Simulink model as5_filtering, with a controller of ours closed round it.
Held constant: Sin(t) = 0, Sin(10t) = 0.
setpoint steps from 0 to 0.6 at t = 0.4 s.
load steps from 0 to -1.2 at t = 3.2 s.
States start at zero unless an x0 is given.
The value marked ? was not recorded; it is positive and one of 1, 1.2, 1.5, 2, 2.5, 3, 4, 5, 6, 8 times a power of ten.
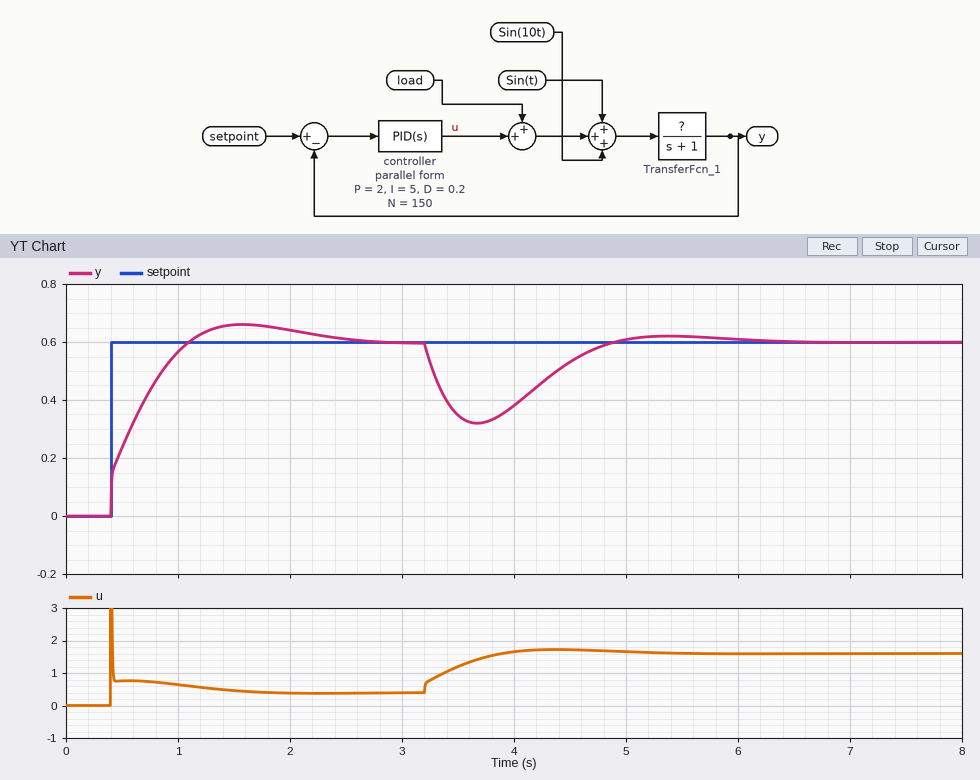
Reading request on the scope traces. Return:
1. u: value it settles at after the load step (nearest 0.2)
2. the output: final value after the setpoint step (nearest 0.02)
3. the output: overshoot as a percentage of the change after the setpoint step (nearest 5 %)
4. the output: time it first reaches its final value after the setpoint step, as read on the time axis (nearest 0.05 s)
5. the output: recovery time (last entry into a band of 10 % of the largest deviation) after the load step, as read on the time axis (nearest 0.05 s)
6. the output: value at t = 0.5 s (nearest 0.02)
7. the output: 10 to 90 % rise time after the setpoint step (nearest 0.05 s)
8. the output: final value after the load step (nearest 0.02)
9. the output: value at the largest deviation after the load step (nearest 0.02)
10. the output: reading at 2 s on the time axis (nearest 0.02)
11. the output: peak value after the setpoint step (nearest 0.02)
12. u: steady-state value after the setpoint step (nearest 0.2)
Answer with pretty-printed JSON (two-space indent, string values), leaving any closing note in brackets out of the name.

{
  "u: value it settles at after the load step": "1.6",
  "the output: final value after the setpoint step": "0.60",
  "the output: overshoot as a percentage of the change after the setpoint step": "10 %",
  "the output: time it first reaches its final value after the setpoint step, as read on the time axis": "1.10 s",
  "the output: recovery time (last entry into a band of 10 % of the largest deviation) after the load step, as read on the time axis": "4.70 s",
  "the output: value at t = 0.5 s": "0.24",
  "the output: 10 to 90 % rise time after the setpoint step": "0.55 s",
  "the output: final value after the load step": "0.60",
  "the output: value at the largest deviation after the load step": "0.32",
  "the output: reading at 2 s on the time axis": "0.64",
  "the output: peak value after the setpoint step": "0.66",
  "u: steady-state value after the setpoint step": "0.4"
}
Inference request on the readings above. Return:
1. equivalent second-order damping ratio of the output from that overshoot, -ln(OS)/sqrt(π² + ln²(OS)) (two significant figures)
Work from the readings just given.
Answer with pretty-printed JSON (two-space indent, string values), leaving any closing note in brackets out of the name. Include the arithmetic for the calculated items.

{
  "equivalent second-order damping ratio of the output from that overshoot, -ln(OS)/sqrt(π² + ln²(OS))": "ln(0.1) = -2.303; 2.303 / sqrt(9.870 + 5.302) = 0.59"
}
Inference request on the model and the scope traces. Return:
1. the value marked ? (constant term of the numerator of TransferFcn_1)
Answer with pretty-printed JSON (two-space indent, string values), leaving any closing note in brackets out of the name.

{
  "the value marked ?": "1.5"
}
